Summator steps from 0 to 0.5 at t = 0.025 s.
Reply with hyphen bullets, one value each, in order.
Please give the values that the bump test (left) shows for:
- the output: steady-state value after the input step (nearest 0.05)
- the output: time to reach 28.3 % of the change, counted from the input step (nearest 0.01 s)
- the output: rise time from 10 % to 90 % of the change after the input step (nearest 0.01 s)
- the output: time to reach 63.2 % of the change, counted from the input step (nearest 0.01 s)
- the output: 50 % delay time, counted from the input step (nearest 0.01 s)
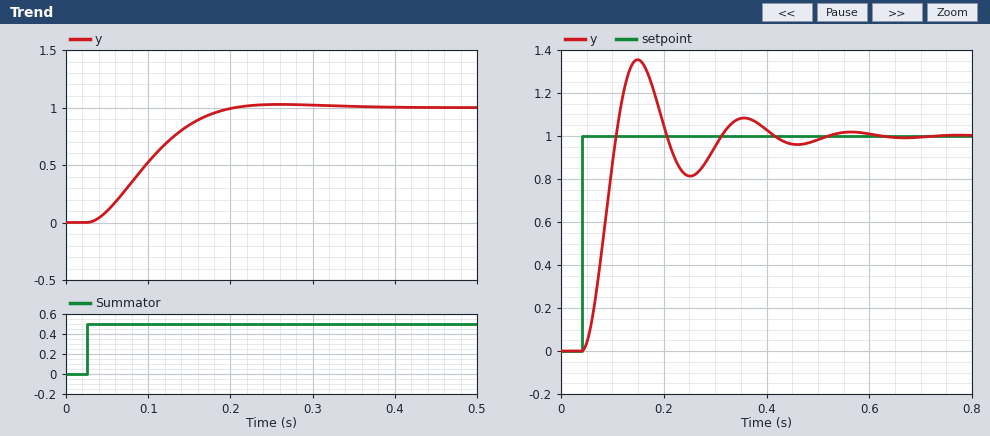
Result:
- 1.00
- 0.05 s
- 0.11 s
- 0.09 s
- 0.07 s
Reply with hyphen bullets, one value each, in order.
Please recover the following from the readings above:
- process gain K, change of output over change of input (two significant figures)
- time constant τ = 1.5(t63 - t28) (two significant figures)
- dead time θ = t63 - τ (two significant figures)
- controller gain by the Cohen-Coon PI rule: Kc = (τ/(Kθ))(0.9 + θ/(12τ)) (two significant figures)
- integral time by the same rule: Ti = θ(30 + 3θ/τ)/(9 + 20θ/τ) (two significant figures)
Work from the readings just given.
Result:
- 2.0
- 0.060 s
- 0.030 s
- 0.94
- 0.050 s
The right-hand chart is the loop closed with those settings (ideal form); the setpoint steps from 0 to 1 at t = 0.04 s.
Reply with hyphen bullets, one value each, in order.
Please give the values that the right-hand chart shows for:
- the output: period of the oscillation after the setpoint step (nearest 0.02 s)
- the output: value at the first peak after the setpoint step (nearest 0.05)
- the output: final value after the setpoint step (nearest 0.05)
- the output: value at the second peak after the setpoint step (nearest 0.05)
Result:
- 0.20 s
- 1.35
- 1.00
- 1.10
